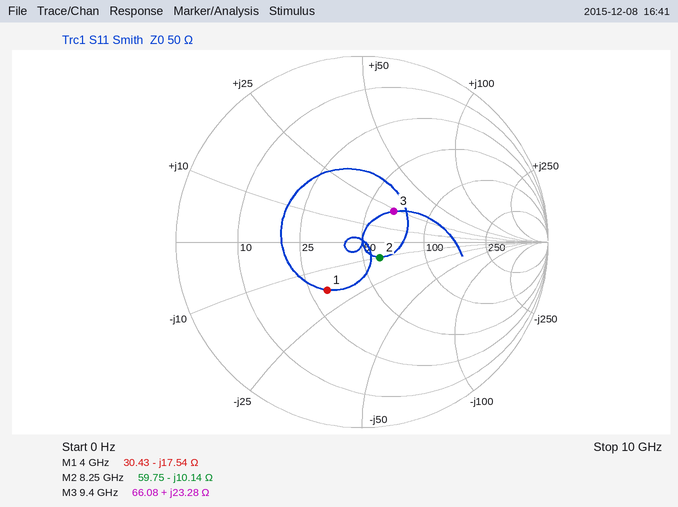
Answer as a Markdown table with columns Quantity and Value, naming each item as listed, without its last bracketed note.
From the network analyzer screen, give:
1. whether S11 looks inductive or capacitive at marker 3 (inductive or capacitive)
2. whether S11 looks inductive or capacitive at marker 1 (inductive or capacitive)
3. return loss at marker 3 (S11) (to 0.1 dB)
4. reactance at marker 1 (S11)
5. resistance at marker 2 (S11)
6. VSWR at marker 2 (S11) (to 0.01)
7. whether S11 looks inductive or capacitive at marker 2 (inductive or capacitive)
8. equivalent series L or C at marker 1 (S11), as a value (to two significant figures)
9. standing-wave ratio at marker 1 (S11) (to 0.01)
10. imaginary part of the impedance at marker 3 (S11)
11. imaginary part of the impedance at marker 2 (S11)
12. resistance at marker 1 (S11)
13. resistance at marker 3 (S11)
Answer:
| Quantity | Value |
|---|---|
| whether S11 looks inductive or capacitive at marker 3 | inductive |
| whether S11 looks inductive or capacitive at marker 1 | capacitive |
| return loss at marker 3 (S11) | 12.4 dB |
| reactance at marker 1 | -17.54 Ω |
| resistance at marker 2 | 59.75 Ω |
| VSWR at marker 2 (S11) | 1.29 |
| whether S11 looks inductive or capacitive at marker 2 | capacitive |
| equivalent series L or C at marker 1 (S11), as a value | 2.3 pF |
| standing-wave ratio at marker 1 (S11) | 1.94 |
| imaginary part of the impedance at marker 3 | +23.28 Ω |
| imaginary part of the impedance at marker 2 | -10.14 Ω |
| resistance at marker 1 | 30.43 Ω |
| resistance at marker 3 | 66.08 Ω |
